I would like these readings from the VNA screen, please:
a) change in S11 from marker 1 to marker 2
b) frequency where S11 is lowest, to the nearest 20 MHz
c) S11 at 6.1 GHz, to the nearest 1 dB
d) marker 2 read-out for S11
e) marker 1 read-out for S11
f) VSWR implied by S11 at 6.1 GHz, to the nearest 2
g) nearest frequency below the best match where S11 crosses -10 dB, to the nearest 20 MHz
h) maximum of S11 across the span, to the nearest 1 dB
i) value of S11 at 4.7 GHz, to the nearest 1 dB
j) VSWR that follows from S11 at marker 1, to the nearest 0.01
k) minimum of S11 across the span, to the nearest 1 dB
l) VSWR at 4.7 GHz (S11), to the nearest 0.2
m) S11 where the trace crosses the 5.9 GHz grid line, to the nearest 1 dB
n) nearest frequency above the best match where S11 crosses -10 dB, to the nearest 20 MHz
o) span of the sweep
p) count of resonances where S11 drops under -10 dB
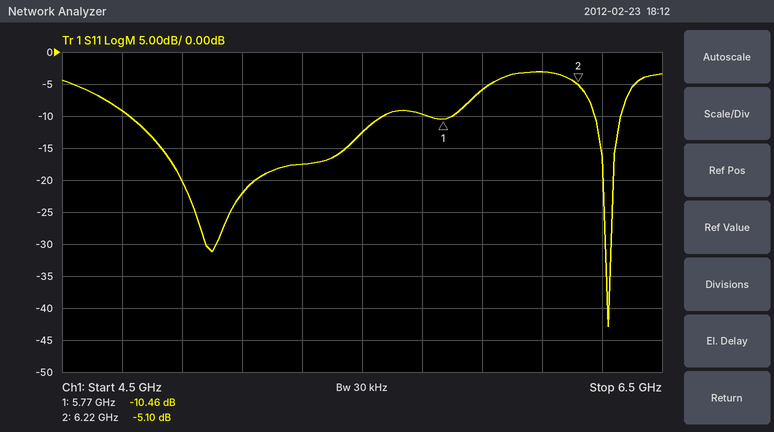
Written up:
5.36 dB
6.32 GHz
-3 dB
-5.10 dB
-10.46 dB
6
6.28 GHz
-3 dB
-9 dB
1.86
-43 dB
2.0
-6 dB
6.36 GHz
2 GHz
2
